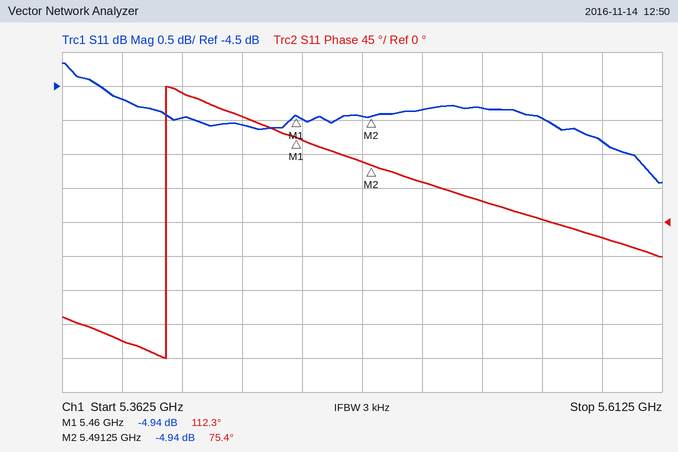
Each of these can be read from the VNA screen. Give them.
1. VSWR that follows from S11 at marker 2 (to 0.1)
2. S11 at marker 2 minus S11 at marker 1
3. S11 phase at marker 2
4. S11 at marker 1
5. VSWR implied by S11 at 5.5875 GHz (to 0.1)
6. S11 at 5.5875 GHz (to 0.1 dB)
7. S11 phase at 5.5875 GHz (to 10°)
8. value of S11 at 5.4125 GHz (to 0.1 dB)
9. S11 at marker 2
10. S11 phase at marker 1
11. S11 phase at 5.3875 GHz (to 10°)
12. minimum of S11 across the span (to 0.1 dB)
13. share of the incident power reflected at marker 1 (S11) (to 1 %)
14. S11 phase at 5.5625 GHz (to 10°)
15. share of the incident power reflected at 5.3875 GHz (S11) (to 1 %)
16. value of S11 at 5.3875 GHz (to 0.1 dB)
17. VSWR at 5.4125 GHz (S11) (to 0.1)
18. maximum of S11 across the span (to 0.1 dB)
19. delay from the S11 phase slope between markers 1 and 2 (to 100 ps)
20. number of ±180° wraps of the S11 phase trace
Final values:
3.6
0.00 dB
75.4°
-4.94 dB
3.4
-5.3 dB
-20°
-5.0 dB
-4.94 dB
112.3°
-160°
-5.9 dB
32 %
0°
34 %
-4.7 dB
3.6
-4.2 dB
3.3 ns
1
